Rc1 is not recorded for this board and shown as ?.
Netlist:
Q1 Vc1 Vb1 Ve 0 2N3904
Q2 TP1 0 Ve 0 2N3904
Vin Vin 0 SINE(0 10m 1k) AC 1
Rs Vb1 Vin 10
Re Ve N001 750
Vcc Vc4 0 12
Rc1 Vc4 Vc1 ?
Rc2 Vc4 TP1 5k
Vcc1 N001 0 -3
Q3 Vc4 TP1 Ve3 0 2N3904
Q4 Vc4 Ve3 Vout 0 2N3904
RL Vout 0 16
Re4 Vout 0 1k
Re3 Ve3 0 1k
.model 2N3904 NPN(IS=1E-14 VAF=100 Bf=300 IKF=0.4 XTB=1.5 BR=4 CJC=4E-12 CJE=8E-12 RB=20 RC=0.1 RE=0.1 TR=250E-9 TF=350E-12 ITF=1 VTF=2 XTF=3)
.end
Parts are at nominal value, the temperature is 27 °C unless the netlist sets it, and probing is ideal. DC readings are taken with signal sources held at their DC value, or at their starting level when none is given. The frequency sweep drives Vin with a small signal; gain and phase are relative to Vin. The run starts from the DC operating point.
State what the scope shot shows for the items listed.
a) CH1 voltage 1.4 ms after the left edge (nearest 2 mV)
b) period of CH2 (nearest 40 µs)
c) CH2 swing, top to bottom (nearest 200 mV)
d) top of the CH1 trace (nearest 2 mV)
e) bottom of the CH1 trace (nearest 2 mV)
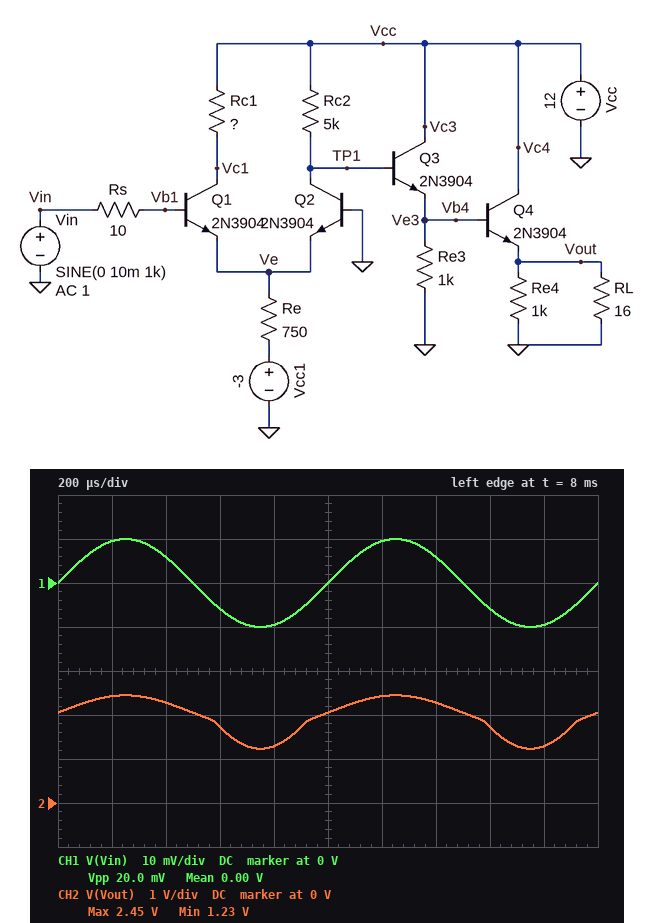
6 mV
1.00 ms
1.2 V
10 mV
-10 mV
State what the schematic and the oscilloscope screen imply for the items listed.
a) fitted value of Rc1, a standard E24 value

9.1 kΩ
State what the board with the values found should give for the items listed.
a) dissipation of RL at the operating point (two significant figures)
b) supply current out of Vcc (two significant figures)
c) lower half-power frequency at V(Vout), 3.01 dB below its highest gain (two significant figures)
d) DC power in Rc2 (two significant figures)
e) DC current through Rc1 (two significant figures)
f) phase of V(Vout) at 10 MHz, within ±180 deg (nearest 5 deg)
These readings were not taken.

260 mW
140 mA
200 kHz
14 mW
1.4 mA
-65 deg
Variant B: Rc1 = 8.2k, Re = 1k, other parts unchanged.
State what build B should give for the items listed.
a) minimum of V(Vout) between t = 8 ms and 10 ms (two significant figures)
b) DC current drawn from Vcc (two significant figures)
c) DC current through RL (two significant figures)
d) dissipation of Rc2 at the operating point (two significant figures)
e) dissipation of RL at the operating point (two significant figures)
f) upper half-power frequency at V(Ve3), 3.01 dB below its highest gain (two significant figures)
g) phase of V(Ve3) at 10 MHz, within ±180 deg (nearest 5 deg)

3.4 V
290 mA
270 mA
7.3 mW
1.2 W
4.4 MHz
-75 deg
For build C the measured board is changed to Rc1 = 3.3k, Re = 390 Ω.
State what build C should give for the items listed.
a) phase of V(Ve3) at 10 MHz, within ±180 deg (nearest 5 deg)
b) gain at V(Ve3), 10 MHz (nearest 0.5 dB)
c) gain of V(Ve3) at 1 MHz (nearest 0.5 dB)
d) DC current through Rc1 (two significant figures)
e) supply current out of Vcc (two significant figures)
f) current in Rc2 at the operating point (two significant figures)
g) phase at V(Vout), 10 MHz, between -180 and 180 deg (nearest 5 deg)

15 deg
-18.5 dB
-26.0 dB
3.3 mA
5.8 mA
2.5 mA
105 deg
